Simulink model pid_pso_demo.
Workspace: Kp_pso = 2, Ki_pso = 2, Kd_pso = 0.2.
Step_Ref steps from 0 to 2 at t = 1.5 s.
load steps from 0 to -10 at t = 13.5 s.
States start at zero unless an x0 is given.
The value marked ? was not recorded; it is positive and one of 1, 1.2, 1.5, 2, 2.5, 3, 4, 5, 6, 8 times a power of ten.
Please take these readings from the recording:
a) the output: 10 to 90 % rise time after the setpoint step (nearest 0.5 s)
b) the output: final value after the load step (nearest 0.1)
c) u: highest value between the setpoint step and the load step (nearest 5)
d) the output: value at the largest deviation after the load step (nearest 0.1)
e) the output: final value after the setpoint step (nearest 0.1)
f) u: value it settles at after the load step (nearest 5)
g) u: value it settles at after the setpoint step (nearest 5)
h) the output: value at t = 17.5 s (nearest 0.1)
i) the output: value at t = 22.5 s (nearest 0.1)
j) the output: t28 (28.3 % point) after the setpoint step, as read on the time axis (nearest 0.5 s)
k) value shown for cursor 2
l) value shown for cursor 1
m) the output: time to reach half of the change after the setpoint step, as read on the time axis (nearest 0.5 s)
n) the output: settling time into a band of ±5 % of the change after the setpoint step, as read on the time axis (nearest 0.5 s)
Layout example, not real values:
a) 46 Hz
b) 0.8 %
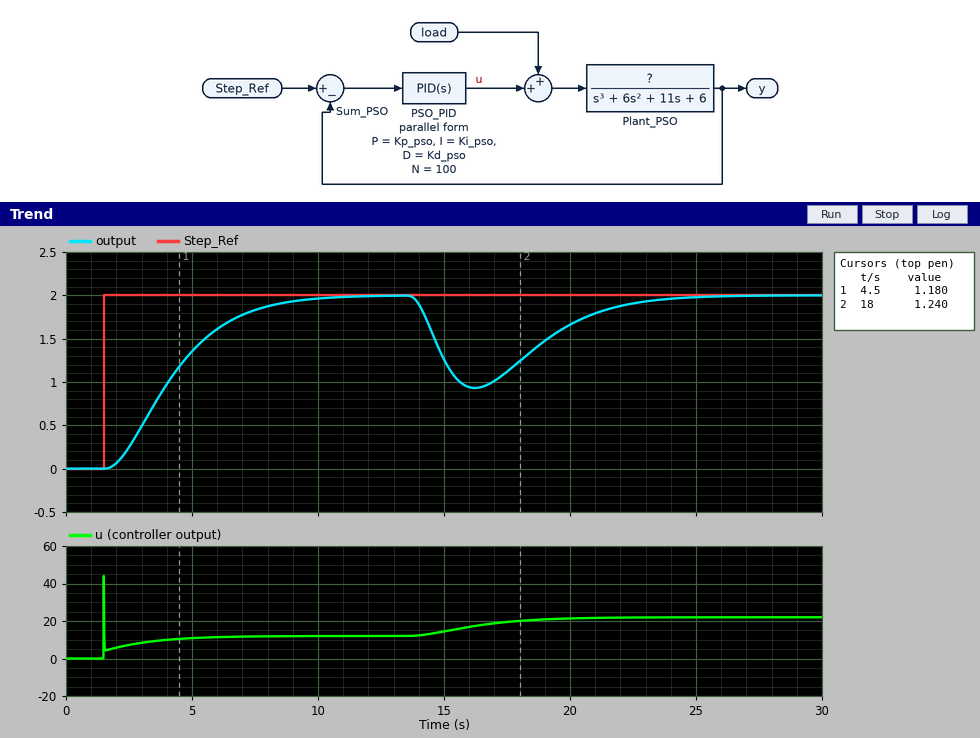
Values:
a) 5.0 s
b) 2.0
c) 45
d) 0.9
e) 2.0
f) 20
g) 10
h) 1.1
i) 1.9
j) 3.0 s
k) 1.240
l) 1.180
m) 4.0 s
n) 8.5 s
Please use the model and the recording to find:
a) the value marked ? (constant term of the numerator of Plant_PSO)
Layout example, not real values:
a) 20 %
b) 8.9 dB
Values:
a) 1
